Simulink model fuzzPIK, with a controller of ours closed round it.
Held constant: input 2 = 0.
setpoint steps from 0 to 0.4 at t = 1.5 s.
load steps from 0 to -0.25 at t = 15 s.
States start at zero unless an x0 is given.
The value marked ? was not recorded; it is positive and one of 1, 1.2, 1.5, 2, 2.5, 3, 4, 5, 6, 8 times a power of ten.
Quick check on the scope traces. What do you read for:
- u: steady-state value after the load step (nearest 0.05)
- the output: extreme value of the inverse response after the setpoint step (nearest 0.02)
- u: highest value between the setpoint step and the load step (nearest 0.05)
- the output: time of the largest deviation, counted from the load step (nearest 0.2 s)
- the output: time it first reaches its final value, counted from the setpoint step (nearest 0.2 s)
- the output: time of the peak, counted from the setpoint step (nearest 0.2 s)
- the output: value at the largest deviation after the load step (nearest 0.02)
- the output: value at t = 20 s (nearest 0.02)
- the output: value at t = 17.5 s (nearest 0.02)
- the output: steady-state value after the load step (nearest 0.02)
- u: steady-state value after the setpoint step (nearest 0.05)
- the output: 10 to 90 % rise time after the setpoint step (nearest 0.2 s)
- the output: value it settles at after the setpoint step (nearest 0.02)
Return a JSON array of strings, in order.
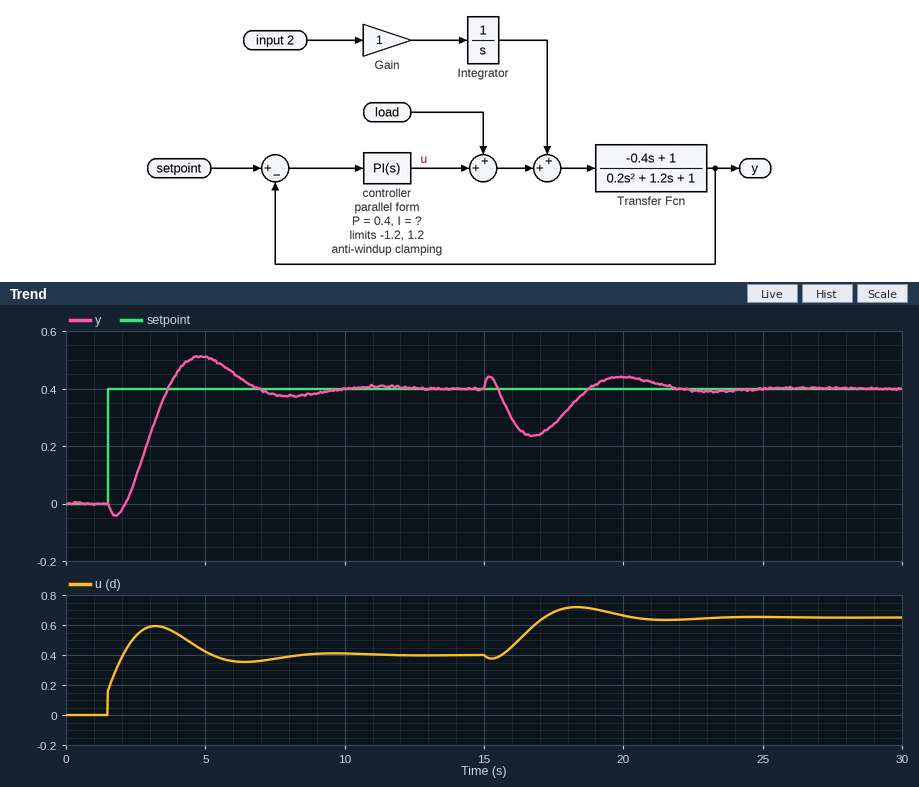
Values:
["0.65", "-0.04", "0.60", "1.8 s", "2.2 s", "3.4 s", "0.24", "0.44", "0.28", "0.40", "0.40", "1.2 s", "0.40"]
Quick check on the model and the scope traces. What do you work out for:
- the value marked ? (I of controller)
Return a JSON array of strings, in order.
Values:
["1"]
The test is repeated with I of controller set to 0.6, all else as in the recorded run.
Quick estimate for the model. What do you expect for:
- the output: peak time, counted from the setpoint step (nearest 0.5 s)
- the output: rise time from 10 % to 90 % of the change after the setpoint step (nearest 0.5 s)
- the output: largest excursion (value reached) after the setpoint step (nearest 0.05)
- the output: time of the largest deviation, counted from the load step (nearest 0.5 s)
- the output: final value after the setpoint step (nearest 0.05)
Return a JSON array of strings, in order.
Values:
["5.0 s", "2.0 s", "0.40", "2.0 s", "0.40"]
